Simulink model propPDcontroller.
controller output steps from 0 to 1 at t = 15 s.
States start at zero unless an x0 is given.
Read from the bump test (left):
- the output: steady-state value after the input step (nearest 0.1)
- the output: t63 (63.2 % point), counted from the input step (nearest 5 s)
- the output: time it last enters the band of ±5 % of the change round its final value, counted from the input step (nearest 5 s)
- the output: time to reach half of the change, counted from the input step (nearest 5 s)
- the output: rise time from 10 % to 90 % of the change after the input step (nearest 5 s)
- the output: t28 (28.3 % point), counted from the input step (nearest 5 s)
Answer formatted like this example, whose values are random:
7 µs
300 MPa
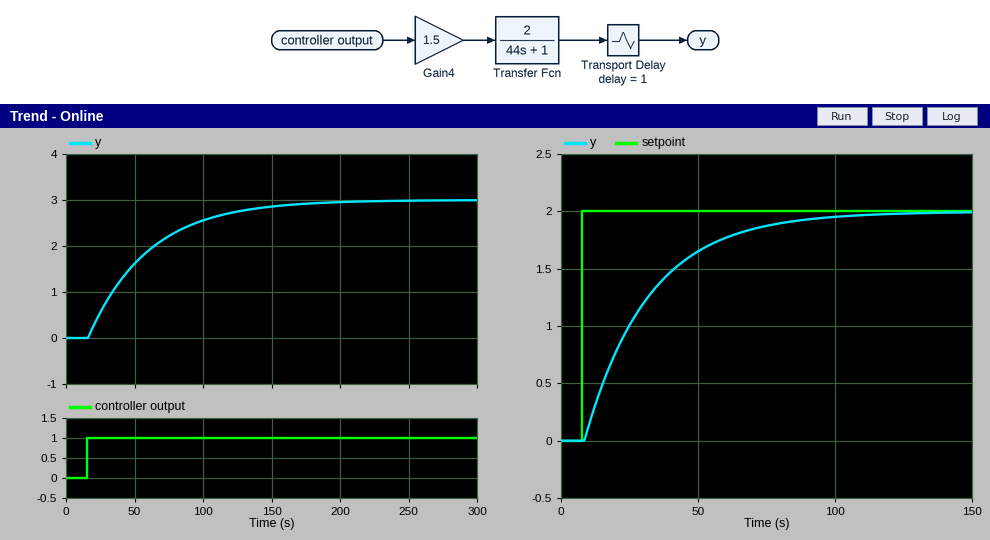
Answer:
3.0
45 s
135 s
30 s
95 s
15 s
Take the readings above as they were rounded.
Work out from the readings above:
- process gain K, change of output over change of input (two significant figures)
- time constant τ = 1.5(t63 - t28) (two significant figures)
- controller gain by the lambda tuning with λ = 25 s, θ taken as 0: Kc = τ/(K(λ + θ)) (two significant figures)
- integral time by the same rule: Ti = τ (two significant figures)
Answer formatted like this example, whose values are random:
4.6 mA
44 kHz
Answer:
3.0
45 s
0.60
45 s
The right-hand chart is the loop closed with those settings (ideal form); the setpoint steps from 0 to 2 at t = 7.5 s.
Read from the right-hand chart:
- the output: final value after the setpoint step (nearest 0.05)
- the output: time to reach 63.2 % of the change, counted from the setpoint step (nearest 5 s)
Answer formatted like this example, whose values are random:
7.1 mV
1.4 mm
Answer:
2.00
25 s
